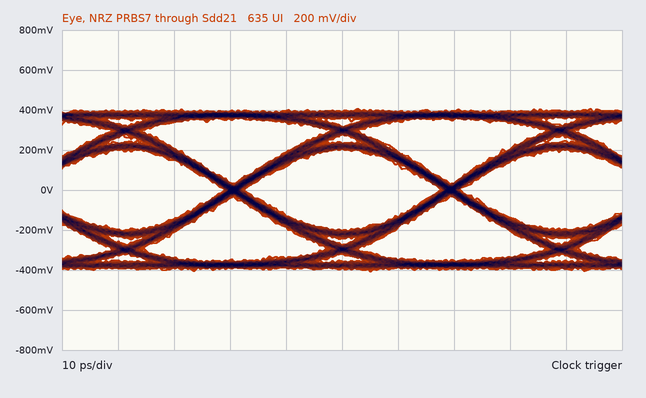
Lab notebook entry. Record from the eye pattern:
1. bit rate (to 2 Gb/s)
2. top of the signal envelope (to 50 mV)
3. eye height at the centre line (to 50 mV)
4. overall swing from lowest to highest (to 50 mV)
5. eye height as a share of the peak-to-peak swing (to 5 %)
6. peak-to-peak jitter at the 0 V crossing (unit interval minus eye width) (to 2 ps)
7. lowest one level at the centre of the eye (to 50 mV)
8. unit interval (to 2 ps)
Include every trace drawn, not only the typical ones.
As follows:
26 Gb/s
400 mV
400 mV
800 mV
50 %
4 ps
200 mV
38 ps
